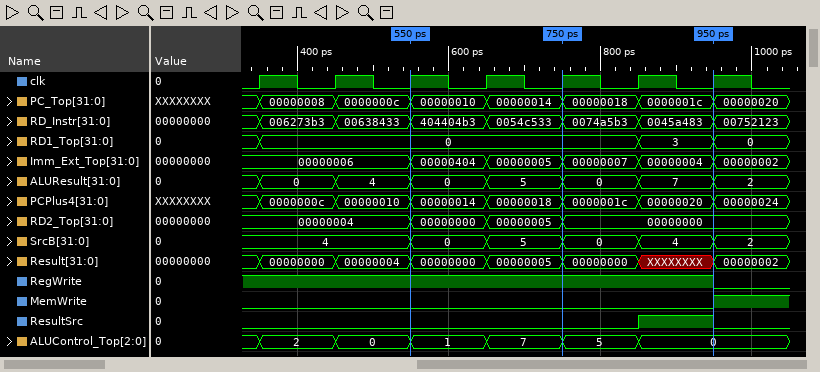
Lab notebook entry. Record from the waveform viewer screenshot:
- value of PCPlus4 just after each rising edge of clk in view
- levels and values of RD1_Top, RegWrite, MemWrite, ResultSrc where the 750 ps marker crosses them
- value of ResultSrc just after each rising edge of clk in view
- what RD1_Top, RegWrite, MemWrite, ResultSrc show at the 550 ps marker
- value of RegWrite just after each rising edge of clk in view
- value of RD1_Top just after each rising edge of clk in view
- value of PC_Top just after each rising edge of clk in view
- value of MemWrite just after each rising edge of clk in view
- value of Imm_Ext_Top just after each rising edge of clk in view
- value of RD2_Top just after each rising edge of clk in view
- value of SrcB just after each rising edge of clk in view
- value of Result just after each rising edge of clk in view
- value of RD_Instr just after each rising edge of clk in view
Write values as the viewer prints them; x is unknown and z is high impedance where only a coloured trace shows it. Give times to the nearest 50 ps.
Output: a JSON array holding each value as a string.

["0000000c, 00000010, 00000014, 00000018, 0000001c, 00000020, 00000024", "RD1_Top=0, RegWrite=1, MemWrite=0, ResultSrc=0", "0 0 0 0 0 1 0", "RD1_Top=0, RegWrite=1, MemWrite=0, ResultSrc=0", "1 1 1 1 1 1 0", "0, 0, 0, 0, 0, 3, 0", "00000008, 0000000c, 00000010, 00000014, 00000018, 0000001c, 00000020", "0 0 0 0 0 0 1", "00000006, 00000006, 00000404, 00000005, 00000007, 00000004, 00000002", "00000004, 00000004, 00000000, 00000005, 00000000, 00000000, 00000000", "4, 4, 0, 5, 0, 4, 2", "00000000, 00000004, 00000000, 00000005, 00000000, XXXXXXXX, 00000002", "006273b3, 00638433, 404404b3, 0054c533, 0074a5b3, 0045a483, 00752123"]
